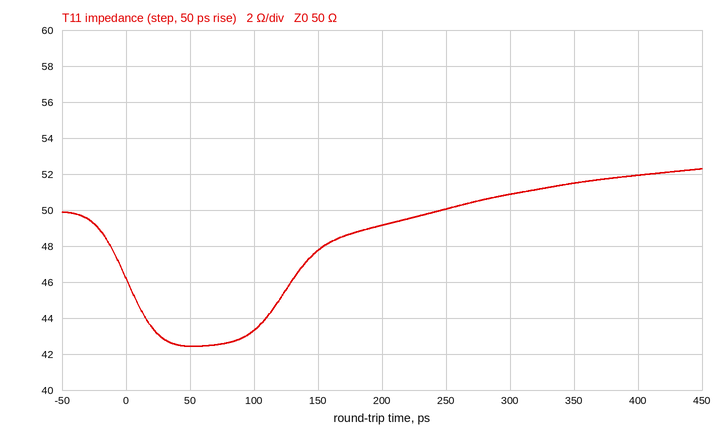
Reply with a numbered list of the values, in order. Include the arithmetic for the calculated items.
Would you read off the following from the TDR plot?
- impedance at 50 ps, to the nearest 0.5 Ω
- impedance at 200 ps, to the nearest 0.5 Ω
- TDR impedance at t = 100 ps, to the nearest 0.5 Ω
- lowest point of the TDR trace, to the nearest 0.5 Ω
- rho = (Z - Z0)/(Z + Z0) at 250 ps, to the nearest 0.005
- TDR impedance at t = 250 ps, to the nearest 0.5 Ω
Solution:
1. 42.5 Ω
2. 49.0 Ω
3. 43.5 Ω
4. 42.5 Ω
5. (50 − 50)/(50 + 50) ≈ 0.000
6. 50.0 Ω
